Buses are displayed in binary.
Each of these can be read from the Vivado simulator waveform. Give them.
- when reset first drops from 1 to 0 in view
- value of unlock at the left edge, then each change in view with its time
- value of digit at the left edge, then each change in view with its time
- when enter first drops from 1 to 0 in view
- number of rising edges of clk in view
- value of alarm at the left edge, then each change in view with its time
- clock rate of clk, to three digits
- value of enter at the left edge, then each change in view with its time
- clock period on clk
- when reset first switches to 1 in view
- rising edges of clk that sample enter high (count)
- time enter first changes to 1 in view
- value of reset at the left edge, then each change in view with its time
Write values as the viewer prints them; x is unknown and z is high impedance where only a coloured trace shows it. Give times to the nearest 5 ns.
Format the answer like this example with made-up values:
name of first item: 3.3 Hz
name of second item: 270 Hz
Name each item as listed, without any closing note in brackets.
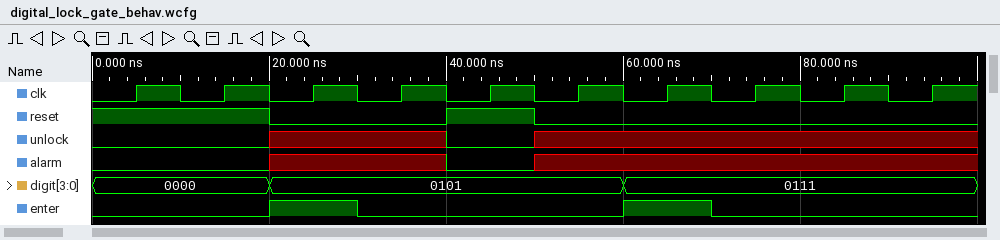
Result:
when reset first drops from 1 to 0 in view: 20 ns
value of unlock at the left edge, then each change in view with its time: 0, x at 20 ns, 0 at 40 ns, x at 50 ns
value of digit at the left edge, then each change in view with its time: 0000, 0101 at 20 ns, 0111 at 60 ns
when enter first drops from 1 to 0 in view: 30 ns
number of rising edges of clk in view: 10
value of alarm at the left edge, then each change in view with its time: 0, x at 20 ns, 0 at 40 ns, x at 50 ns
clock rate of clk, to three digits: 100 MHz
value of enter at the left edge, then each change in view with its time: 0, 1 at 20 ns, 0 at 30 ns, 1 at 60 ns, 0 at 70 ns
clock period on clk: 10 ns
when reset first switches to 1 in view: 40 ns
rising edges of clk that sample enter high: 2
time enter first changes to 1 in view: 20 ns
value of reset at the left edge, then each change in view with its time: 1, 0 at 20 ns, 1 at 40 ns, 0 at 50 ns
